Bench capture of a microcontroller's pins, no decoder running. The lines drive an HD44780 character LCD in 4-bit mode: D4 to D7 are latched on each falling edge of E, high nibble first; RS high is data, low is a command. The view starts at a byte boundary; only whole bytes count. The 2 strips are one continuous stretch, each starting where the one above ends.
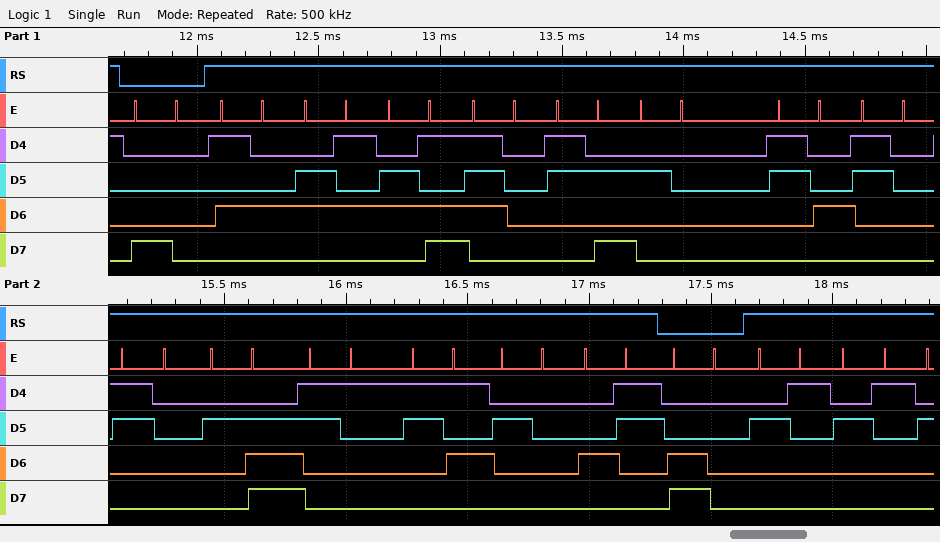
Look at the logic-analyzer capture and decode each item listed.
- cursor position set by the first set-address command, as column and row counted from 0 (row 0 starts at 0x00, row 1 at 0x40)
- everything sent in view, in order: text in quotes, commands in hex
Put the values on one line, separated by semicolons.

column 0, row 0; 0x80 "Temp: 400.15 C" 0xC0 "!!"
